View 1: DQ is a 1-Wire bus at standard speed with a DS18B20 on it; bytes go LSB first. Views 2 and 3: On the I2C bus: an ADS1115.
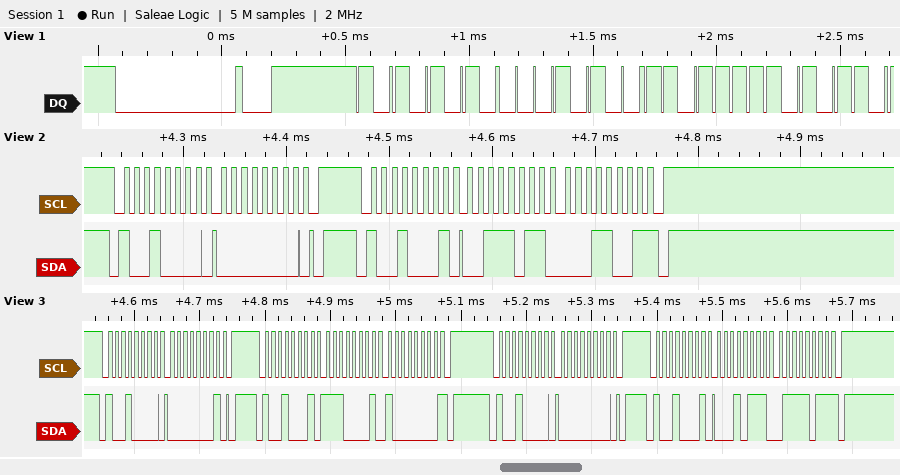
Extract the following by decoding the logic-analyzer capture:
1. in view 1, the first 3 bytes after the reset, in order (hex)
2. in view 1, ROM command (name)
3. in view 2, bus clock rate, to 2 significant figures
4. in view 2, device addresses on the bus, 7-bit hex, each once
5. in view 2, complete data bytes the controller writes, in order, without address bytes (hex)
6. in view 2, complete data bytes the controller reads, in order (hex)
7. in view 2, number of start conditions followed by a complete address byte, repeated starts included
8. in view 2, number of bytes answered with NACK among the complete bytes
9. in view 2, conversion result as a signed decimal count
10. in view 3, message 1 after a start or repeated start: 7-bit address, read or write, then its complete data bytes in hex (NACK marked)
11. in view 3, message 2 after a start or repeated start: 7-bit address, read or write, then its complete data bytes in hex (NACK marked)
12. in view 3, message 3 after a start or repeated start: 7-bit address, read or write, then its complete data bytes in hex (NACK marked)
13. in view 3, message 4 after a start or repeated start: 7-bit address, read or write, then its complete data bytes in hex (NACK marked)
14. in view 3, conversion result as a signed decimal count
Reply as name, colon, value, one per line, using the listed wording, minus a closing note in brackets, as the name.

in view 1, the first 3 bytes after the reset, in order: 55 28 FB
in view 1, ROM command: Match ROM
in view 2, bus clock rate, to 2 significant figures: 100 kHz
in view 2, device addresses on the bus, 7-bit hex, each once: 0x48
in view 2, complete data bytes the controller writes, in order, without address bytes: 00
in view 2, complete data bytes the controller reads, in order: 3B 19
in view 2, number of start conditions followed by a complete address byte, repeated starts included: 2
in view 2, number of bytes answered with NACK among the complete bytes: 1
in view 2, conversion result as a signed decimal count: 15129
in view 3, message 1 after a start or repeated start: 7-bit address, read or write, then its complete data bytes in hex: 0x48 write: 01
in view 3, message 2 after a start or repeated start: 7-bit address, read or write, then its complete data bytes in hex: 0x48 read: E1 80 NACK
in view 3, message 3 after a start or repeated start: 7-bit address, read or write, then its complete data bytes in hex: 0x48 write: 00
in view 3, message 4 after a start or repeated start: 7-bit address, read or write, then its complete data bytes in hex: 0x48 read: 17 7B NACK
in view 3, conversion result as a signed decimal count: 6011
